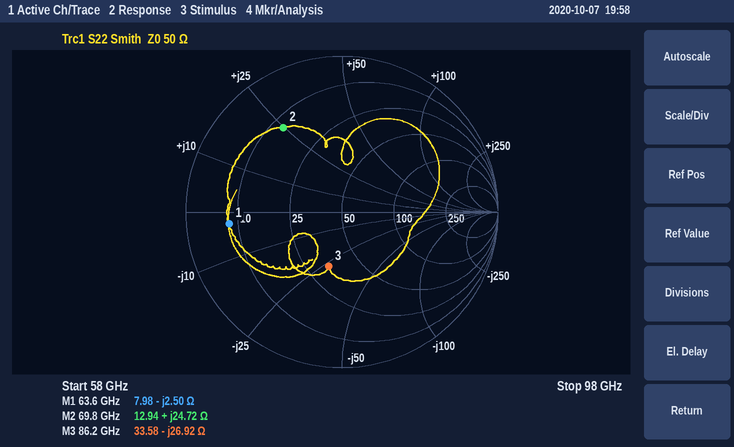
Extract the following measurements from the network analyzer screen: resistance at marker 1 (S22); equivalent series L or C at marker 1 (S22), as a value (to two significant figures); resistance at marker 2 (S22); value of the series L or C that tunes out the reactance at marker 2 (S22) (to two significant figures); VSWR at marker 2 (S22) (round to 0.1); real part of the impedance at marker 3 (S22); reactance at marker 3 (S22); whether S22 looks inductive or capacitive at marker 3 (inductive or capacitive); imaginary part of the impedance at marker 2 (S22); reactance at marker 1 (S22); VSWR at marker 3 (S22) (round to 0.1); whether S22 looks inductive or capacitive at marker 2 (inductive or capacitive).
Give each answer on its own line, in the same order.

7.98 Ω
1.00 pF
12.94 Ω
92 fF
4.9
33.58 Ω
-26.92 Ω
capacitive
+24.72 Ω
-2.50 Ω
2.1
inductive
